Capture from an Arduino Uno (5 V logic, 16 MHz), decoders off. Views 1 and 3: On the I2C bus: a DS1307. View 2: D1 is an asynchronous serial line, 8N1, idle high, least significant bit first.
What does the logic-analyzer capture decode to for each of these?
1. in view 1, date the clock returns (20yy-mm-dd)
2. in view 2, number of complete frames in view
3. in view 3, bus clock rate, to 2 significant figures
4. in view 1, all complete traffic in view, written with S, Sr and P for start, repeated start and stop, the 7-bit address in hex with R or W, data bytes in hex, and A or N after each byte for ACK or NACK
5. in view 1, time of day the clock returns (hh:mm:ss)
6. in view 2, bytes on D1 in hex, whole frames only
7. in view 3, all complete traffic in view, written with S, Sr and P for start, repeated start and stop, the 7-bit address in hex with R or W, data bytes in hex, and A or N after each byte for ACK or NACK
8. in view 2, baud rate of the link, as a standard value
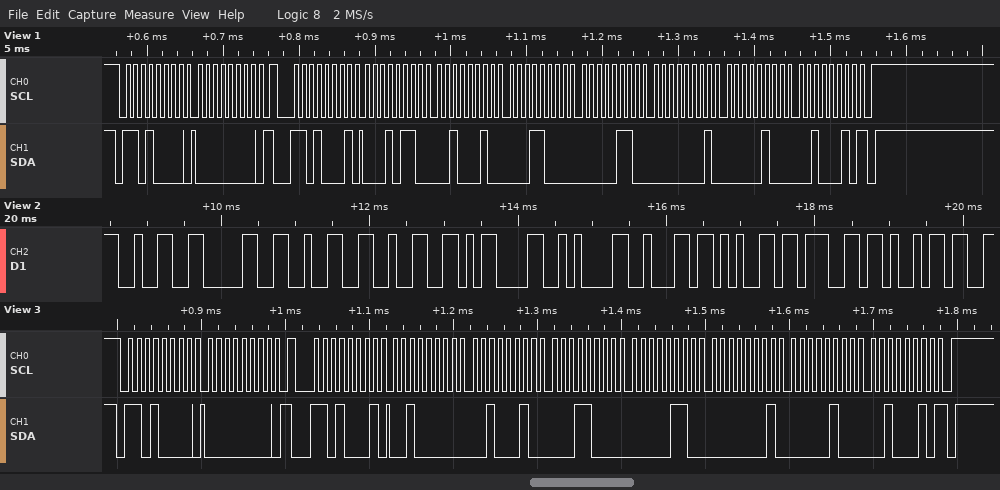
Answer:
2022-04-01
10
100 kHz
S 68W A 00 A Sr 68R A 16 A 22 A 18 A 06 A 01 A 04 A 22 N P
18:22:16
32 30 32 32 0D 0A 62 65 67 69
S 68W A 00 A Sr 68R A 20 A 22 A 18 A 06 A 01 A 04 A 22 N P
9600 baud
